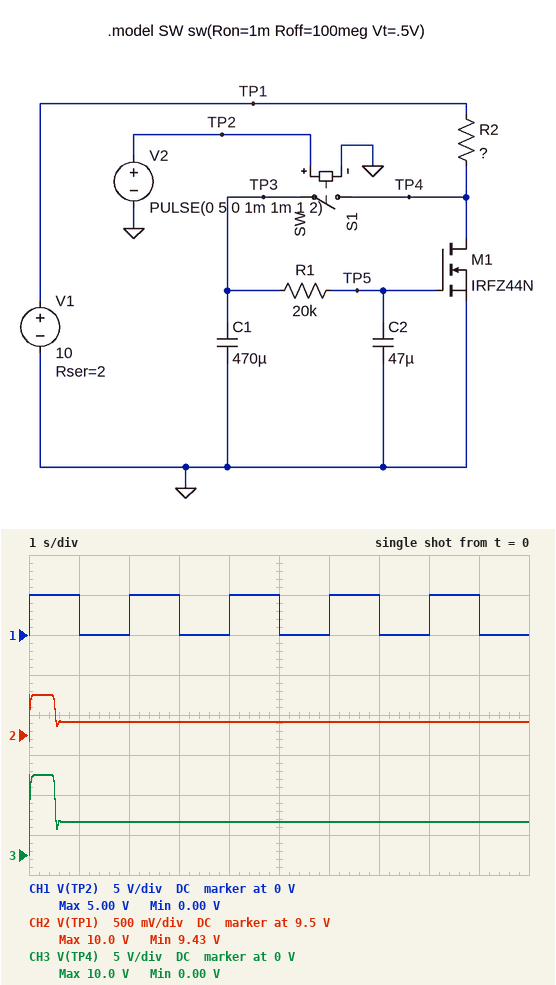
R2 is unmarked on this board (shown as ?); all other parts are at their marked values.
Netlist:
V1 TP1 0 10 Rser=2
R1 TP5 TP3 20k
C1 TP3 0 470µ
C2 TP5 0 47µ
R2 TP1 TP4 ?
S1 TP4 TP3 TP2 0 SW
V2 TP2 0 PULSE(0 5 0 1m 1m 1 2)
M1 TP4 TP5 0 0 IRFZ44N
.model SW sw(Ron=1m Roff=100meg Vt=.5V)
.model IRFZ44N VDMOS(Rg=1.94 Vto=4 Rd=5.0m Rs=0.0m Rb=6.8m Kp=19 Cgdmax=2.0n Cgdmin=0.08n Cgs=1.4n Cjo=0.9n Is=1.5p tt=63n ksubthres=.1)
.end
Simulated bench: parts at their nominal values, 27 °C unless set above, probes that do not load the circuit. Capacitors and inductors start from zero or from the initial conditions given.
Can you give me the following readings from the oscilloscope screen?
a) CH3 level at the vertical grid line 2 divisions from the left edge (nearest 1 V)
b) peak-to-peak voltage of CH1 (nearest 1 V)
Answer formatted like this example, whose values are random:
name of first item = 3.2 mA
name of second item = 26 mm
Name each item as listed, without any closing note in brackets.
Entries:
CH3 level at the vertical grid line 2 divisions from the left edge = 4 V
peak-to-peak voltage of CH1 = 5 V
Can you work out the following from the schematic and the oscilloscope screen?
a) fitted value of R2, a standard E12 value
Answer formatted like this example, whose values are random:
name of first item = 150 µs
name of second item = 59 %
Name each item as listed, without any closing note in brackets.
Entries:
fitted value of R2, a standard E12 value = 33 Ω
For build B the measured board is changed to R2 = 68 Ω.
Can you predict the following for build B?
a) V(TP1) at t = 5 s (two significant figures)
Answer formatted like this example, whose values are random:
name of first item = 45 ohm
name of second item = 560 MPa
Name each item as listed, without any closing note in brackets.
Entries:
V(TP1) at t = 5 s = 9.8 V
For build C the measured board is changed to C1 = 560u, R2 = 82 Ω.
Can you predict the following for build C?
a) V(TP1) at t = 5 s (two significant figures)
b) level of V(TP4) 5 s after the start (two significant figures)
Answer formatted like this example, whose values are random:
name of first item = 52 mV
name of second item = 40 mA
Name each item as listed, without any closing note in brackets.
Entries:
V(TP1) at t = 5 s = 9.9 V
level of V(TP4) 5 s after the start = 4.0 V
